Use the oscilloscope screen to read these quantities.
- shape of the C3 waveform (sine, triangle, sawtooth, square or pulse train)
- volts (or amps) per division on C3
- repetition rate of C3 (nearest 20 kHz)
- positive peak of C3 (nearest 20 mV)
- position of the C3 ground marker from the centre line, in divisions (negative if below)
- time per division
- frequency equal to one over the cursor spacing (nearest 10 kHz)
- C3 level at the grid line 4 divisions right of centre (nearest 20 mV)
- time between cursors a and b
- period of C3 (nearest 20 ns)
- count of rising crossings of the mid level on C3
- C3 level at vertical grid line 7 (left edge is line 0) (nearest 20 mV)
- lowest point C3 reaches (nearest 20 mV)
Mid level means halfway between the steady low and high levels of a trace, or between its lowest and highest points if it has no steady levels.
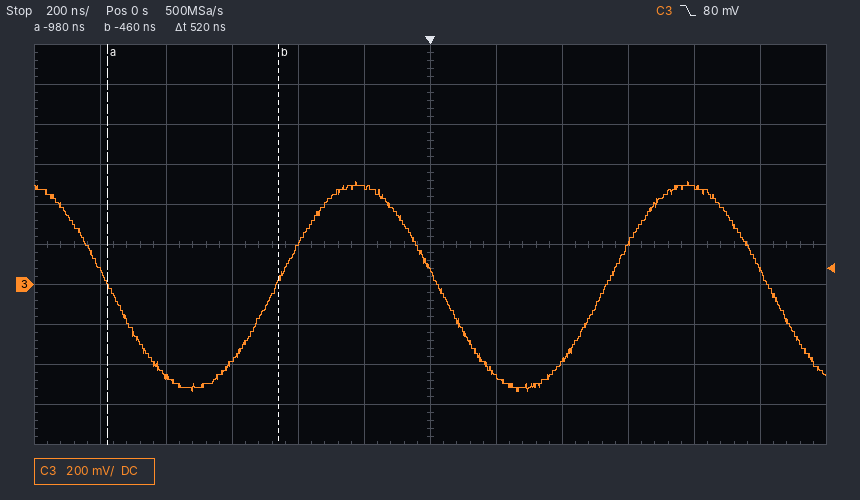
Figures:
sine
200 mV
1.00 MHz
520 mV
-1.0 div
200 ns
1.92 MHz
480 mV
520 ns
1.00 µs
2
-460 mV
-540 mV
